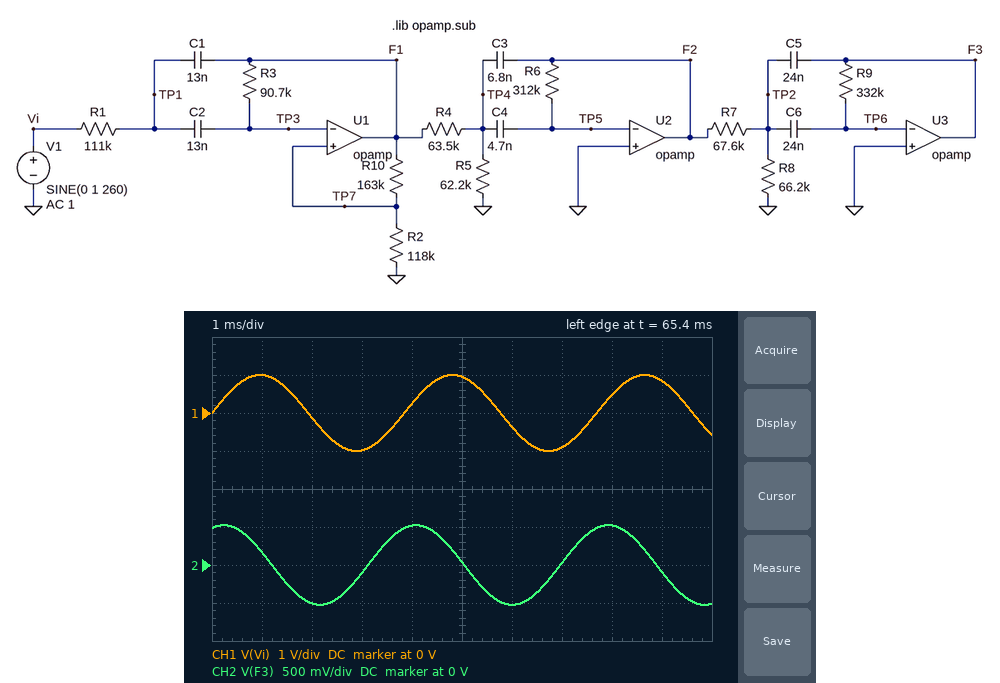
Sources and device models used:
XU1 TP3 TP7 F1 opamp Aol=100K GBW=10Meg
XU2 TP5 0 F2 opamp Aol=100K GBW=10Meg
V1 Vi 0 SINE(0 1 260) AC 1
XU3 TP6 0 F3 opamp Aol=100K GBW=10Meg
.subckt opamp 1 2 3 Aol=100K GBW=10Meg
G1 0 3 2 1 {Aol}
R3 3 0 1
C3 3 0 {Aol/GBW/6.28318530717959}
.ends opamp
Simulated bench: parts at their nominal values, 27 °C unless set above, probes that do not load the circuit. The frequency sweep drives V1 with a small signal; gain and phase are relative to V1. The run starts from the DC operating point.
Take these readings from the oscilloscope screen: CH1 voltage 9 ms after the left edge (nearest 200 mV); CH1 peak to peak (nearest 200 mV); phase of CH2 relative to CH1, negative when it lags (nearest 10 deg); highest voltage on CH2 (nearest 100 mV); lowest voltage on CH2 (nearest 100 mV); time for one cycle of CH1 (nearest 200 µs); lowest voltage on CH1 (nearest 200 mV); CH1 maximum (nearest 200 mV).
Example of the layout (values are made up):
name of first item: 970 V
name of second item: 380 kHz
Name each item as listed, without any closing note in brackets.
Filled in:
CH1 voltage 9 ms after the left edge: 800 mV
CH1 peak to peak: 2.0 V
phase of CH2 relative to CH1, negative when it lags: 70 deg
highest voltage on CH2: 500 mV
lowest voltage on CH2: -500 mV
time for one cycle of CH1: 3.8 ms
lowest voltage on CH1: -1.0 V
CH1 maximum: 1.0 V
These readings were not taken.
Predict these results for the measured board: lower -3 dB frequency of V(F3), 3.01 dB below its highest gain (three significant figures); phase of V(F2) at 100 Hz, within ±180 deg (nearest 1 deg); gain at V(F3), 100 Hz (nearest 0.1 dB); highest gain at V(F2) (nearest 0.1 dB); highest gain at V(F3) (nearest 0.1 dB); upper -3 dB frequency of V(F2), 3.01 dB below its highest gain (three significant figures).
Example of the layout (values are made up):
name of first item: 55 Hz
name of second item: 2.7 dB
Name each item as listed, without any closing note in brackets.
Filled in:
lower -3 dB frequency of V(F3), 3.01 dB below its highest gain: 59.1 Hz
phase of V(F2) at 100 Hz, within ±180 deg: 90 deg
gain at V(F3), 100 Hz: -3.6 dB
highest gain at V(F2): 2.4 dB
highest gain at V(F3): -3.5 dB
upper -3 dB frequency of V(F2), 3.01 dB below its highest gain: 342 Hz
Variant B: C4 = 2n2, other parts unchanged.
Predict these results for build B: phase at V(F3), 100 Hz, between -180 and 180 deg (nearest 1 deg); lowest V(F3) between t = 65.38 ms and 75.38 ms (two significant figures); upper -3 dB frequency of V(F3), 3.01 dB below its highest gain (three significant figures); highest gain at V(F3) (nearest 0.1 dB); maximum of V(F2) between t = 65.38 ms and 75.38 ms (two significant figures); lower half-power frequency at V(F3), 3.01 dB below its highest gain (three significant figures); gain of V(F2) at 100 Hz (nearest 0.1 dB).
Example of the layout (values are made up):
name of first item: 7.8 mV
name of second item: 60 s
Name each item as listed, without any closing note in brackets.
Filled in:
phase at V(F3), 100 Hz, between -180 and 180 deg: -143 deg
lowest V(F3) between t = 65.38 ms and 75.38 ms: -200 mV
upper -3 dB frequency of V(F3), 3.01 dB below its highest gain: 223 Hz
highest gain at V(F3): -10.5 dB
maximum of V(F2) between t = 65.38 ms and 75.38 ms: 500 mV
lower half-power frequency at V(F3), 3.01 dB below its highest gain: 58.6 Hz
gain of V(F2) at 100 Hz: -13.3 dB
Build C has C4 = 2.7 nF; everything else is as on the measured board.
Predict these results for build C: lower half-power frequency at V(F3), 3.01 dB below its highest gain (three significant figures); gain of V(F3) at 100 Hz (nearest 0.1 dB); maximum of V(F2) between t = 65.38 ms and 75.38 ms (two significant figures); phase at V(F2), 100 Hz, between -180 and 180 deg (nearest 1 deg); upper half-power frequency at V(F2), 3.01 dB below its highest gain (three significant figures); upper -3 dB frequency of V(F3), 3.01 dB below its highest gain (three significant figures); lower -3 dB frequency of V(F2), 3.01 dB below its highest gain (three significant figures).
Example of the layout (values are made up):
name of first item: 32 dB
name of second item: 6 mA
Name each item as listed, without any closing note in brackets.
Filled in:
lower half-power frequency at V(F3), 3.01 dB below its highest gain: 58.7 Hz
gain of V(F3) at 100 Hz: -8.8 dB
maximum of V(F2) between t = 65.38 ms and 75.38 ms: 650 mV
phase at V(F2), 100 Hz, between -180 and 180 deg: 93 deg
upper half-power frequency at V(F2), 3.01 dB below its highest gain: 450 Hz
upper -3 dB frequency of V(F3), 3.01 dB below its highest gain: 252 Hz
lower -3 dB frequency of V(F2), 3.01 dB below its highest gain: 187 Hz
